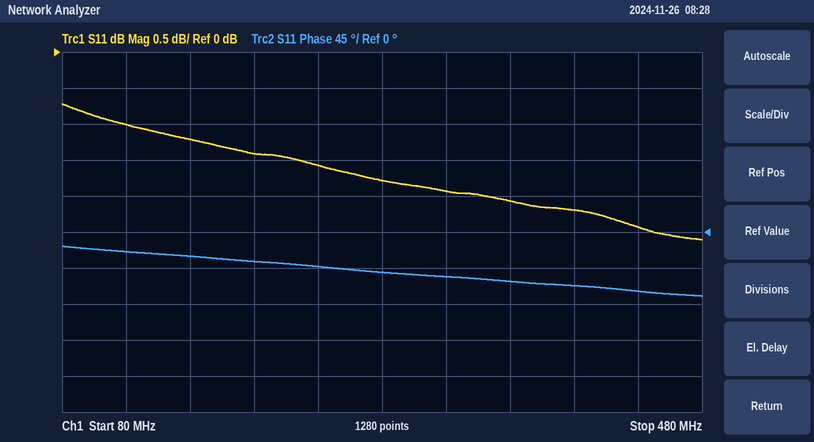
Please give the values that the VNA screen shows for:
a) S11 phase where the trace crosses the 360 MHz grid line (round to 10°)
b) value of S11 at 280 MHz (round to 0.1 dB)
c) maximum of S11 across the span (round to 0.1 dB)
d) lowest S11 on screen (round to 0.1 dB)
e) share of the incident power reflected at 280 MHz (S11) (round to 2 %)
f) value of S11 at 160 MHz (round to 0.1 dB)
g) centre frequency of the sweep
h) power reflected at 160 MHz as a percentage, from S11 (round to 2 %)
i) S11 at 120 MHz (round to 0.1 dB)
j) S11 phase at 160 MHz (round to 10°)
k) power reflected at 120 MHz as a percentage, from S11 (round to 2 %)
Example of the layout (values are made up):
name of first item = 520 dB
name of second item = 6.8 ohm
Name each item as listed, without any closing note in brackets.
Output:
S11 phase where the trace crosses the 360 MHz grid line = -60°
value of S11 at 280 MHz = -1.8 dB
maximum of S11 across the span = -0.7 dB
lowest S11 on screen = -2.6 dB
share of the incident power reflected at 280 MHz (S11) = 66 %
value of S11 at 160 MHz = -1.2 dB
centre frequency of the sweep = 280 MHz
power reflected at 160 MHz as a percentage, from S11 = 76 %
S11 at 120 MHz = -1.0 dB
S11 phase at 160 MHz = -30°
power reflected at 120 MHz as a percentage, from S11 = 80 %
